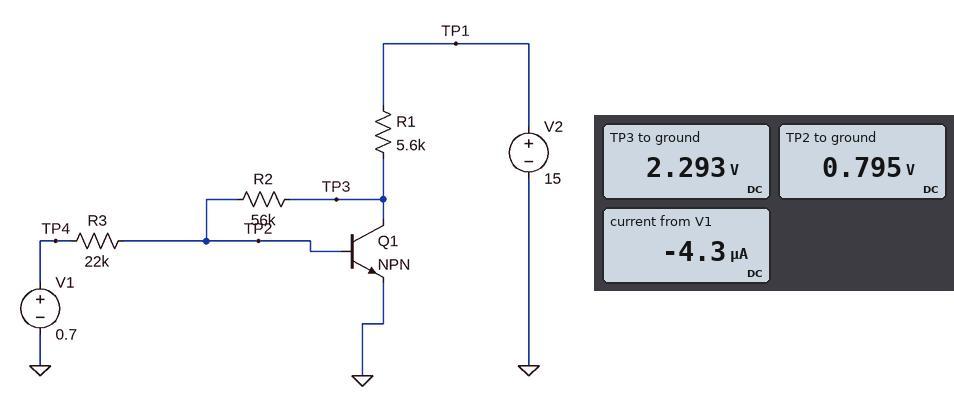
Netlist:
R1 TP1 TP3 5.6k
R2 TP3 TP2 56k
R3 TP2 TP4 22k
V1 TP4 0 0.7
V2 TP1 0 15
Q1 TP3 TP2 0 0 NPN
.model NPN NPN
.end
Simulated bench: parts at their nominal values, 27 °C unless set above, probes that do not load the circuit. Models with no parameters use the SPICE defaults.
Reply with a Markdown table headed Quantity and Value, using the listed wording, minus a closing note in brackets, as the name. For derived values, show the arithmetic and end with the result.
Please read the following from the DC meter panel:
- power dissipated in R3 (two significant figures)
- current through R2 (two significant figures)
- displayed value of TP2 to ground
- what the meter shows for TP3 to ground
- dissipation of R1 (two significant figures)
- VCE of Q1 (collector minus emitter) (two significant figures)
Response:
| Quantity | Value |
|---|---|
| power dissipated in R3 | (795 mV - 700 mV)^2 / 22 kΩ = 410 nW |
| current through R2 | (2.293 V - 795 mV) / 56 kΩ = 27 µA |
| displayed value of TP2 to ground | 0.795 V |
| what the meter shows for TP3 to ground | 2.293 V |
| dissipation of R1 | (15 V - 2.293 V)^2 / 5.6 kΩ = 29 mW |
| VCE of Q1 (collector minus emitter) | 2.293 V = 2.3 V |
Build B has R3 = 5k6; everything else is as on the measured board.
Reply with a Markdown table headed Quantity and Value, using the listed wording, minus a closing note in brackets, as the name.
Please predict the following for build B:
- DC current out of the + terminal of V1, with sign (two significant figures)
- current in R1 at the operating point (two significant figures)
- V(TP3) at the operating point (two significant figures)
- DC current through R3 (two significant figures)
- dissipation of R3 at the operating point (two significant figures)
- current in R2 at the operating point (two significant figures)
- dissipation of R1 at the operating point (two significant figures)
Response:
| Quantity | Value |
|---|---|
| DC current out of the + terminal of V1, with sign | -17 µA |
| current in R1 at the operating point | 2.2 mA |
| V(TP3) at the operating point | 2.9 V |
| DC current through R3 | 17 µA |
| dissipation of R3 at the operating point | 1.6 µW |
| current in R2 at the operating point | 38 µA |
| dissipation of R1 at the operating point | 26 mW |
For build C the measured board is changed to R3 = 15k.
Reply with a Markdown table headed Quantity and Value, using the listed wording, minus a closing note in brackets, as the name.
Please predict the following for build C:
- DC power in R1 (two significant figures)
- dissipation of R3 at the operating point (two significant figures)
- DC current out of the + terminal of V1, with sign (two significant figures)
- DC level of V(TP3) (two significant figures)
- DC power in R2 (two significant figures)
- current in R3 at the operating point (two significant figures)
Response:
| Quantity | Value |
|---|---|
| DC power in R1 | 28 mW |
| dissipation of R3 at the operating point | 600 nW |
| DC current out of the + terminal of V1, with sign | -6.3 µA |
| DC level of V(TP3) | 2.4 V |
| DC power in R2 | 46 µW |
| current in R3 at the operating point | 6.3 µA |
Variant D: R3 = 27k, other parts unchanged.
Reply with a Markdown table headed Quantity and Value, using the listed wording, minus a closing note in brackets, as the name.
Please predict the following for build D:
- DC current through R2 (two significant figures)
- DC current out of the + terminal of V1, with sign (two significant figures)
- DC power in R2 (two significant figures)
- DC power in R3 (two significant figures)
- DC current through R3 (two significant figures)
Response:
| Quantity | Value |
|---|---|
| DC current through R2 | 26 µA |
| DC current out of the + terminal of V1, with sign | -3.5 µA |
| DC power in R2 | 38 µW |
| DC power in R3 | 340 nW |
| DC current through R3 | 3.5 µA |
